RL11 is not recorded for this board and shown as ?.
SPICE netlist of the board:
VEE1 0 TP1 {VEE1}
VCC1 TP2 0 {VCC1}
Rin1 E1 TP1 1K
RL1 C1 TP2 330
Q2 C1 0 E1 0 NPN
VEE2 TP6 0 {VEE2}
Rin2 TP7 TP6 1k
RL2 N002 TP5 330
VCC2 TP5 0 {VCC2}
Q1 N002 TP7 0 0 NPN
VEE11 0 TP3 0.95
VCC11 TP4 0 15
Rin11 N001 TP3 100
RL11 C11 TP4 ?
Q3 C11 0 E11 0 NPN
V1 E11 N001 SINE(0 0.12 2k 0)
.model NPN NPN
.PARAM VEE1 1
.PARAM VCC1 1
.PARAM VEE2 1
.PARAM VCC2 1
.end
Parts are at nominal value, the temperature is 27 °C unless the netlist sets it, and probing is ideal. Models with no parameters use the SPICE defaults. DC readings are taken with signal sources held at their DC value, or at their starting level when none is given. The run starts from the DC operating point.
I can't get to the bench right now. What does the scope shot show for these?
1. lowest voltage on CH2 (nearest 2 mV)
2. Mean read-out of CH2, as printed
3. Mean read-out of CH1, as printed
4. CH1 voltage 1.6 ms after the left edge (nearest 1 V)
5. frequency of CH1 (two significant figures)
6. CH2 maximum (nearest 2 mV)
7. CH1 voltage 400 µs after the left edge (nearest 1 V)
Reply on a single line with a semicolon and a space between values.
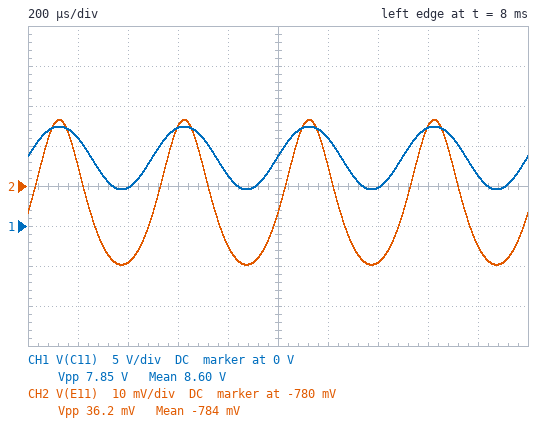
-800 mV; -784 mV; 8.60 V; 12 V; 2.0 kHz; -764 mV; 5 V
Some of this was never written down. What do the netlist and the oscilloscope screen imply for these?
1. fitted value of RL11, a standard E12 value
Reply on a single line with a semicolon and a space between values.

3.9 kΩ
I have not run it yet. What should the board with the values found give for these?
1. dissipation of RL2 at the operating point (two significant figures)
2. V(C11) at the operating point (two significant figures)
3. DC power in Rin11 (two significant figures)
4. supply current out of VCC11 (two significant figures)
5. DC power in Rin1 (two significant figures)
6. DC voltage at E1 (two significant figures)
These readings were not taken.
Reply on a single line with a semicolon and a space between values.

2.6 mW; 8.7 V; 270 µW; 1.6 mA; 68 µW; -740 mV
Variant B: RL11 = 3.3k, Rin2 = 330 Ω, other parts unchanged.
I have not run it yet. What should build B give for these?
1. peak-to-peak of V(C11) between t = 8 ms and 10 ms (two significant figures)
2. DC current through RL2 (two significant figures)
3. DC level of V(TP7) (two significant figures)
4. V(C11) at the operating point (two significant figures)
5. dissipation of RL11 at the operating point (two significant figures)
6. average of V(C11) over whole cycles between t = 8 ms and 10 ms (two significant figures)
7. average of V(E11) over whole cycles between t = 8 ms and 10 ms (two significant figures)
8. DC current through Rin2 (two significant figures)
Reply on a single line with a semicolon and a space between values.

6.7 V; 2.9 mA; 810 mV; 9.7 V; 8.6 mW; 9.6 V; -780 mV; 580 µA
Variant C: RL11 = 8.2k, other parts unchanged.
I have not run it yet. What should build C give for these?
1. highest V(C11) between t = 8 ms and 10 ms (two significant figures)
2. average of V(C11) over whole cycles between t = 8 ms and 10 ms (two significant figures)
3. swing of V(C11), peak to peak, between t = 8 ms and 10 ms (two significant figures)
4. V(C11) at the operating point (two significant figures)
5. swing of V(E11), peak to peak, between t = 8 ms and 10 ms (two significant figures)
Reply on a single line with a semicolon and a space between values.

9.6 V; 3.2 V; 10 V; 1.7 V; 42 mV
